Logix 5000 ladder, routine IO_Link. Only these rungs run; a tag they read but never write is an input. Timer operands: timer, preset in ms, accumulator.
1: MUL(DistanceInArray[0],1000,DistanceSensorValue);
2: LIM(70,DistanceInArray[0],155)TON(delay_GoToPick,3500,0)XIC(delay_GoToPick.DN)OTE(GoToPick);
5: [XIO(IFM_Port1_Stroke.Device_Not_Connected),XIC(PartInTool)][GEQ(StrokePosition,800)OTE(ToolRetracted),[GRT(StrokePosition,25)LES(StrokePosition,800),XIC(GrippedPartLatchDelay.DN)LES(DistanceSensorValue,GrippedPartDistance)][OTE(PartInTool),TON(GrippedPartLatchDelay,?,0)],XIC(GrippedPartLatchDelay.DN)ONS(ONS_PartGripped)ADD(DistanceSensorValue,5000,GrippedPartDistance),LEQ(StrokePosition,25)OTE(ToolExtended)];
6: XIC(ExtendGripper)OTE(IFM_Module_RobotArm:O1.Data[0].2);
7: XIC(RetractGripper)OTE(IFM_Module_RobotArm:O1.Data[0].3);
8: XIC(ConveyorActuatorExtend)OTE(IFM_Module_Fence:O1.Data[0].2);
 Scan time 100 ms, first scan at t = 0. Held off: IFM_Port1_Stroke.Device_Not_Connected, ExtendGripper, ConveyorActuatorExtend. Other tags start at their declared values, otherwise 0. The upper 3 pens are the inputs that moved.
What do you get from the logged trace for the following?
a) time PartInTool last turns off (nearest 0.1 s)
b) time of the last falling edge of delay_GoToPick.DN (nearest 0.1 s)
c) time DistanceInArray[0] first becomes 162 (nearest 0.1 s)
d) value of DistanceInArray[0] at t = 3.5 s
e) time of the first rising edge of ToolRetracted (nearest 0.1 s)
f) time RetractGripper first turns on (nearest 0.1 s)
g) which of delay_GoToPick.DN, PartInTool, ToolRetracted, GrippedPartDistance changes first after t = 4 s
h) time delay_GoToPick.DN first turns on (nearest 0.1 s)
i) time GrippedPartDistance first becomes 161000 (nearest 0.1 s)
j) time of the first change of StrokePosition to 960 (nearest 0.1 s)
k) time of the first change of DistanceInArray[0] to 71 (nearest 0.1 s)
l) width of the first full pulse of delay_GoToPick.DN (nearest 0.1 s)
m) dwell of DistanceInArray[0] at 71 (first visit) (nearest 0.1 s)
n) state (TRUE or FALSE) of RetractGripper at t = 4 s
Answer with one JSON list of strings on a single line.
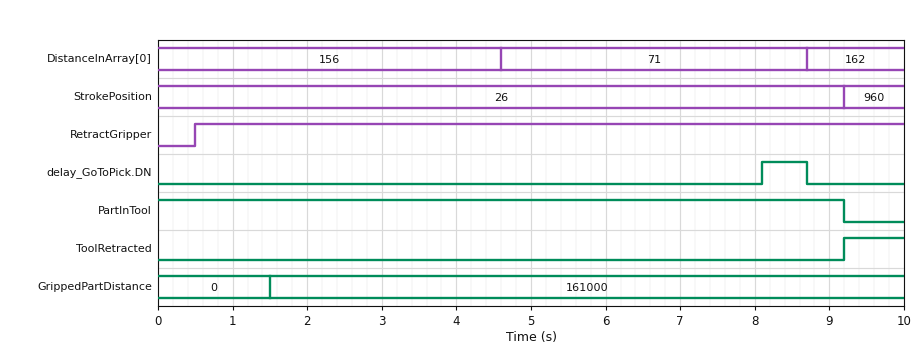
["9.2 s", "8.7 s", "8.7 s", "156", "9.2 s", "0.5 s", "delay_GoToPick.DN", "8.1 s", "1.5 s", "9.2 s", "4.6 s", "0.6 s", "4.1 s", "TRUE"]
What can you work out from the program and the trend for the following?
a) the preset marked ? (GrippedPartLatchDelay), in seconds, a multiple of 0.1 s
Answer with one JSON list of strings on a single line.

["1.5 s"]
